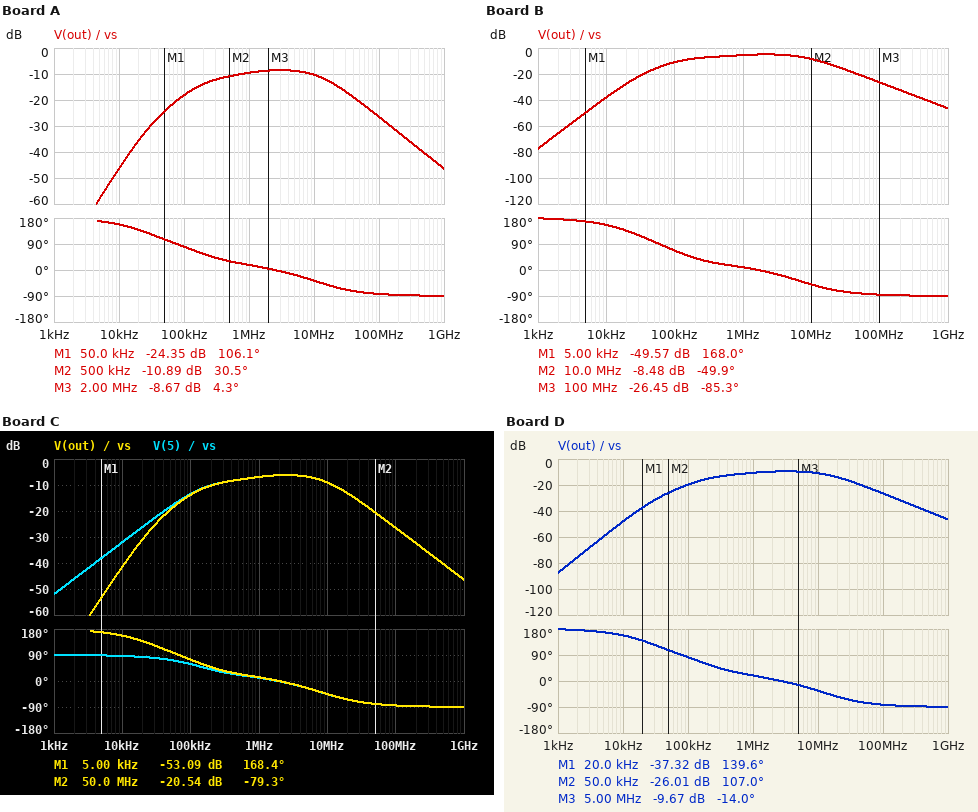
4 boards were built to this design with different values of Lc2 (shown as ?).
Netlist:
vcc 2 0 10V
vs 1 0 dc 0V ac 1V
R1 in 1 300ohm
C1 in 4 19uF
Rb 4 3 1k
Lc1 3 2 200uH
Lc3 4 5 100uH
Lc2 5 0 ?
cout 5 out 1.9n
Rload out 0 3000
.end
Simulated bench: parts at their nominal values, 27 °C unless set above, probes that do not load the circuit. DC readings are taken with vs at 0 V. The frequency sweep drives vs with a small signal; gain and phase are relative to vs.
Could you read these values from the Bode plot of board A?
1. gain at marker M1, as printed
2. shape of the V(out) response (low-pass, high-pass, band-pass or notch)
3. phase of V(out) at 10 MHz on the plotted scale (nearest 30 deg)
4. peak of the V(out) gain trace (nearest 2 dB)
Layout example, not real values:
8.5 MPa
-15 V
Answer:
-24.35 dB
band-pass
-30 deg
-8 dB
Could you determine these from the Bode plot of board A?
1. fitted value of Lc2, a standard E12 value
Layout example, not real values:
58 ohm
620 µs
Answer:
68 µH
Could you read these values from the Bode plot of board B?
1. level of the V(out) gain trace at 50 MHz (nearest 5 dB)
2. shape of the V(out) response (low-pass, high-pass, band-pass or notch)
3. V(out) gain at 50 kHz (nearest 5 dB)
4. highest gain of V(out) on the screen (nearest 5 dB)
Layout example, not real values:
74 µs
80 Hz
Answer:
-20 dB
band-pass
-15 dB
-5 dB
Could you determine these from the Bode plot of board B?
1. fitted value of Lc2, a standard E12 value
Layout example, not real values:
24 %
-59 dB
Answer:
180 µH
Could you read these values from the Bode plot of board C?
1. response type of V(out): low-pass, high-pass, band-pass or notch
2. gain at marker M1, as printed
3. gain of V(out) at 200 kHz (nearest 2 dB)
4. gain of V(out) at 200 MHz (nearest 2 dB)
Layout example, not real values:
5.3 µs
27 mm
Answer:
band-pass
-53.09 dB
-10 dB
-32 dB
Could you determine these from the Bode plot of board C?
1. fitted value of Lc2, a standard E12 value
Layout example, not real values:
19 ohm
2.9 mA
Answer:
120 µH
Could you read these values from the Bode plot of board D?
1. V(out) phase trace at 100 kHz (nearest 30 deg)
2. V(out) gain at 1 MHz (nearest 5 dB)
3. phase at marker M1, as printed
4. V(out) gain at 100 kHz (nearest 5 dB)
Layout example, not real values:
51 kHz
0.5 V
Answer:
90 deg
-10 dB
139.6 deg
-20 dB
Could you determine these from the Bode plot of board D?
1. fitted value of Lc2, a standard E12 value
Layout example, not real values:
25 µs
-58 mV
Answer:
56 µH
